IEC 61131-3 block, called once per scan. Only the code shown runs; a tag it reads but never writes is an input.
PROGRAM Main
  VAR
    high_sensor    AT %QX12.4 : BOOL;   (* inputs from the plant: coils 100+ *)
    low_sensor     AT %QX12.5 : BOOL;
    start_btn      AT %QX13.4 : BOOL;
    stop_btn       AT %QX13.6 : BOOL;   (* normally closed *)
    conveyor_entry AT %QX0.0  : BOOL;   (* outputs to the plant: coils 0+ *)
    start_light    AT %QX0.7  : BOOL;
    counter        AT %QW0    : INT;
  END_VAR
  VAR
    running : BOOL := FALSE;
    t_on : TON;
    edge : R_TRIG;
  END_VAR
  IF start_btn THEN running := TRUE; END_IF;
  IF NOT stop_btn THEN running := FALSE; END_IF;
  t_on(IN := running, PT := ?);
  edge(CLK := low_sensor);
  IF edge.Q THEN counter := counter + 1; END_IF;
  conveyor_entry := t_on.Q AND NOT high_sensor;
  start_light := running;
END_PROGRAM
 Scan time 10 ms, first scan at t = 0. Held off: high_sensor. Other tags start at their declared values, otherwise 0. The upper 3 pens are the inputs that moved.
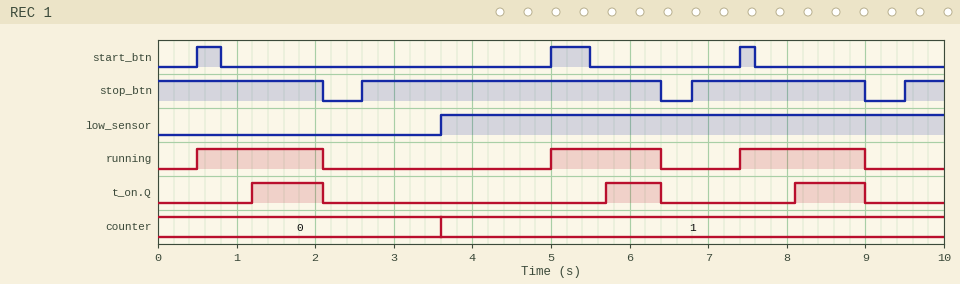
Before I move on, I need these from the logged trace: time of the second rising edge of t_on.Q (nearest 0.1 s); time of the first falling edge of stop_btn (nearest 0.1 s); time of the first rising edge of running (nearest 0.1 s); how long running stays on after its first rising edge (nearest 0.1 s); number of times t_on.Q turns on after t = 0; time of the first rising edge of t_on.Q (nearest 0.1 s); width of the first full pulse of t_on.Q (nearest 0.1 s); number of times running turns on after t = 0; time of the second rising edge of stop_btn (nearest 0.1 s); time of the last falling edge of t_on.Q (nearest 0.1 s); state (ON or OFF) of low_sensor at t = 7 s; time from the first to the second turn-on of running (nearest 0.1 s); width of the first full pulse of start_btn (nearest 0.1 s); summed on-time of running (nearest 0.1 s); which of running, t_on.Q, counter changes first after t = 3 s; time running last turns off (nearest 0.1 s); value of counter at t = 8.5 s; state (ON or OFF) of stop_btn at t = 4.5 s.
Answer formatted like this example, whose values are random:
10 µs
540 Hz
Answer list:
5.7 s
2.1 s
0.5 s
1.6 s
3
1.2 s
0.9 s
3
6.8 s
9.0 s
ON
4.5 s
0.3 s
4.6 s
counter
9.0 s
1
ON
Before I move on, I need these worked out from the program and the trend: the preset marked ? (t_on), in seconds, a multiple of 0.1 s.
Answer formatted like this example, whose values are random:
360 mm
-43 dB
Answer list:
0.7 s
